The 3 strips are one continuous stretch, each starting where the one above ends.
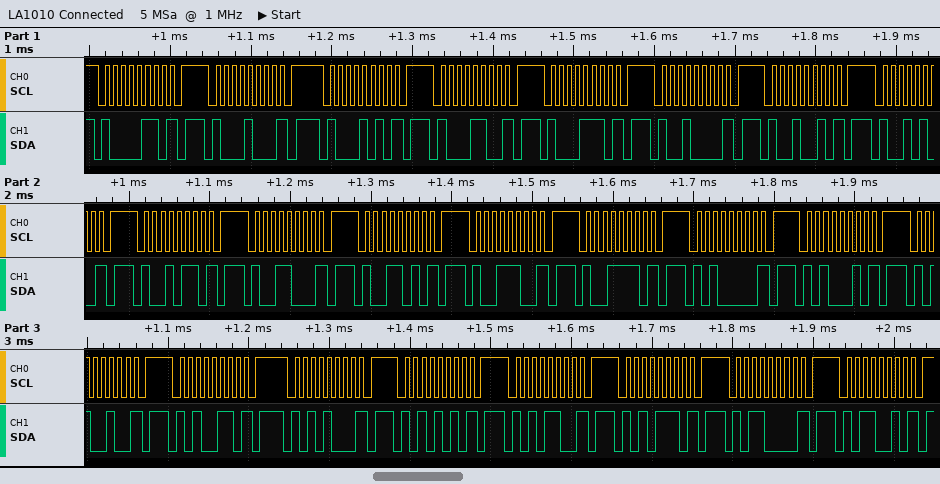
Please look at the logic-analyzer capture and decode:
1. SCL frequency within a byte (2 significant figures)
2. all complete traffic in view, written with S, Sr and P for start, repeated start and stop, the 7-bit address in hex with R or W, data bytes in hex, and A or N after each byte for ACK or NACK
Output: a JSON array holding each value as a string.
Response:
["100 kHz", "S 43W N P S 44W N P S 45W N P S 46W N P S 47W N P S 48W N P S 49W N P S 4AW N P S 4BW N P S 4CW N P S 4DW N P S 4EW N P S 4FW N P S 50W N P S 51W N P S 52W N P S 53W N P S 54W N P S 55W N P S 56W N P S 57W N P S 58W N P S 59W N P"]
